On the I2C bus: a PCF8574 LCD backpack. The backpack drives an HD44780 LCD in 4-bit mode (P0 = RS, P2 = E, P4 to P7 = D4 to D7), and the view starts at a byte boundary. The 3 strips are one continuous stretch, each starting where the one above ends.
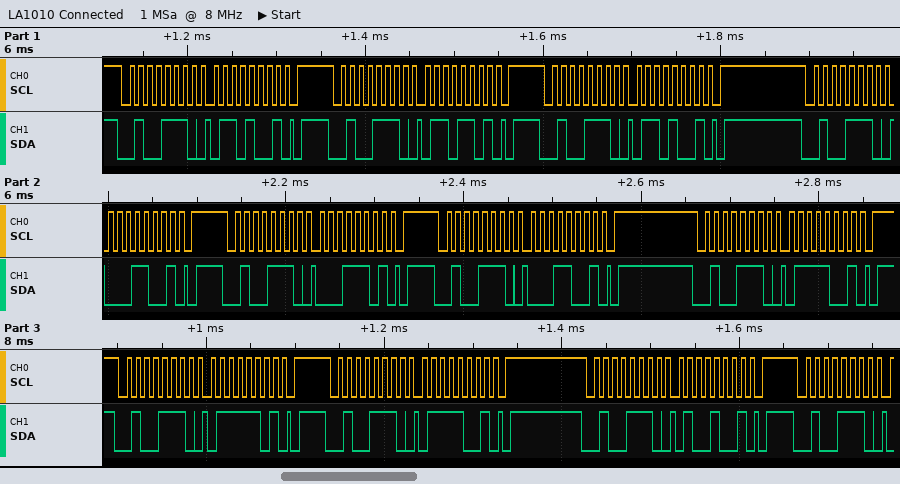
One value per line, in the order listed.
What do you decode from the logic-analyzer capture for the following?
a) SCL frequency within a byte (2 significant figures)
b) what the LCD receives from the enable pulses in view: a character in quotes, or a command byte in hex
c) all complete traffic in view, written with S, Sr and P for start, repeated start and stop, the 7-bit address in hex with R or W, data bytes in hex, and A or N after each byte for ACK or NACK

100 kHz
'a'
S 27W A 69 A P S 27W A 6D A P S 27W A 69 A P S 27W A 19 A P S 27W A 1D A P S 27W A 19 A P S 27W A 79 A P S 27W A 7D A P S 27W A 79 A P S 27W A 49 A P S 27W A
